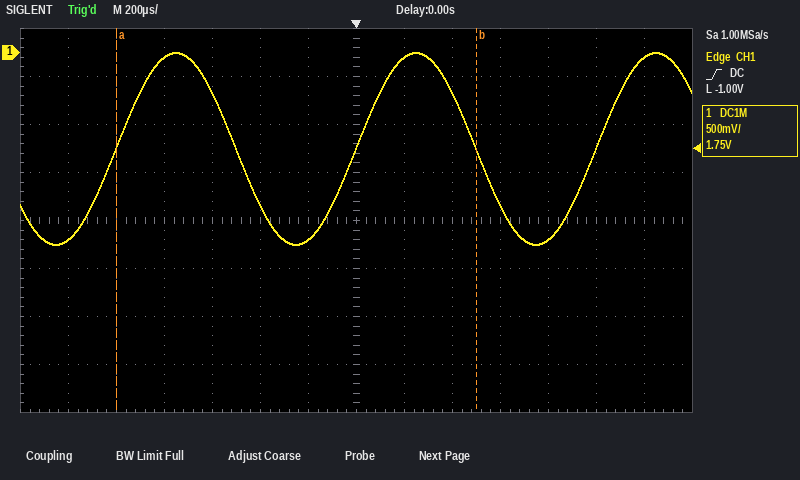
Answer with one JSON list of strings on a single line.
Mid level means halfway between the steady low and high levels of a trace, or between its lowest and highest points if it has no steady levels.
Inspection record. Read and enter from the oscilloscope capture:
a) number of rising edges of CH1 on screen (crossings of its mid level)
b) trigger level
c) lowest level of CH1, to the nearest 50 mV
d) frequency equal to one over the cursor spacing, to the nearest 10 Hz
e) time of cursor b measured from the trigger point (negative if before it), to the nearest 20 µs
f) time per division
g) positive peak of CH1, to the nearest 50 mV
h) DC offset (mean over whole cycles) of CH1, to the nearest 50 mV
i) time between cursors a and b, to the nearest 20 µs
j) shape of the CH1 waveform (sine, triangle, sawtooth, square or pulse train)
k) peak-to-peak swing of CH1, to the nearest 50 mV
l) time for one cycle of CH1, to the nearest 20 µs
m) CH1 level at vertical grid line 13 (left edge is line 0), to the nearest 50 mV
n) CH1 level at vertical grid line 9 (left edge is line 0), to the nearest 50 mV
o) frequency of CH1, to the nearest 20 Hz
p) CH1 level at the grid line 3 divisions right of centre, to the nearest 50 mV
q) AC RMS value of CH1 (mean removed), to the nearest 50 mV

["3", "-1.00 V", "-2.00 V", "670 Hz", "+500 µs", "200 µs", "0 mV", "-1.00 V", "1.50 ms", "sine", "2.00 V", "1.00 ms", "-50 mV", "-400 mV", "1.00 kHz", "-1.60 V", "700 mV"]
